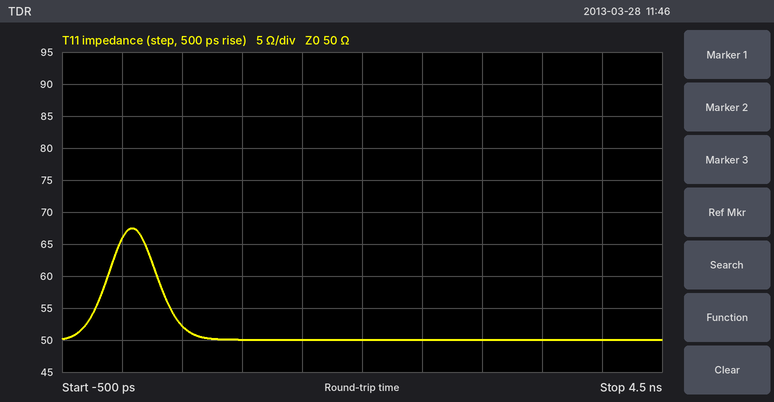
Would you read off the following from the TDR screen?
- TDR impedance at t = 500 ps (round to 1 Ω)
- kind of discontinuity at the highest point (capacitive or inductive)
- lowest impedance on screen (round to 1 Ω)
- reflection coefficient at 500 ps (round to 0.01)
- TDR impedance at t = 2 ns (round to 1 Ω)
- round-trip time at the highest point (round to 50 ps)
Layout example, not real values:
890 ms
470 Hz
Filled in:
52 Ω
inductive
50 Ω
+0.02
50 Ω
100 ps
